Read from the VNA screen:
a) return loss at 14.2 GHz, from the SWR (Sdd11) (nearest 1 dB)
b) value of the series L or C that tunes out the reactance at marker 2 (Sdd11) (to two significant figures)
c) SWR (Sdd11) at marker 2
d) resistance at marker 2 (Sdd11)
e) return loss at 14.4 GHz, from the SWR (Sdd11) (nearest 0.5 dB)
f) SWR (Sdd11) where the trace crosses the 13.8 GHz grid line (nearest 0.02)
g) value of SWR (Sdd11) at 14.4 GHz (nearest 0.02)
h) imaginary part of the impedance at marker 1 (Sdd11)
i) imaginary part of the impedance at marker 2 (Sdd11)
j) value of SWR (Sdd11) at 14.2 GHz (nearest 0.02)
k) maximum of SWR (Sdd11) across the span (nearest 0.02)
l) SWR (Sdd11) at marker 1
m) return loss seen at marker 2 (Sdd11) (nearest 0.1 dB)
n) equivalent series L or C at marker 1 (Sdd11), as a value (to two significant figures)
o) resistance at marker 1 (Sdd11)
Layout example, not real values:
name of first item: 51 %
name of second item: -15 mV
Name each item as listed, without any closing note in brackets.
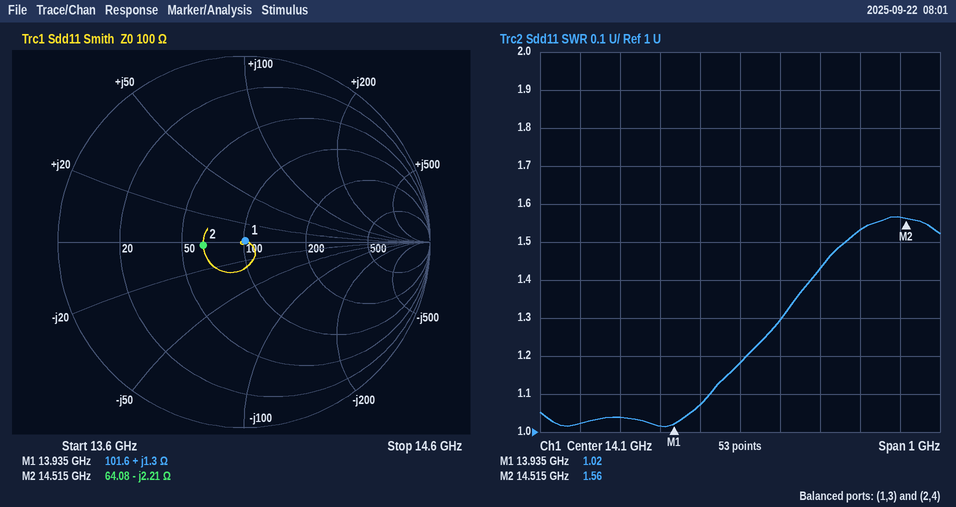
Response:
return loss at 14.2 GHz, from the SWR (Sdd11): 18 dB
value of the series L or C that tunes out the reactance at marker 2 (Sdd11): 24 pH
SWR (Sdd11) at marker 2: 1.56
resistance at marker 2: 64.08 Ω
return loss at 14.4 GHz, from the SWR (Sdd11): 13.5 dB
SWR (Sdd11) where the trace crosses the 13.8 GHz grid line: 1.04
value of SWR (Sdd11) at 14.4 GHz: 1.54
imaginary part of the impedance at marker 1: +1.3 Ω
imaginary part of the impedance at marker 2: -2.21 Ω
value of SWR (Sdd11) at 14.2 GHz: 1.30
maximum of SWR (Sdd11) across the span: 1.56
SWR (Sdd11) at marker 1: 1.02
return loss seen at marker 2 (Sdd11): 13.2 dB
equivalent series L or C at marker 1 (Sdd11), as a value: 15 pH
resistance at marker 1: 101.6 Ω
